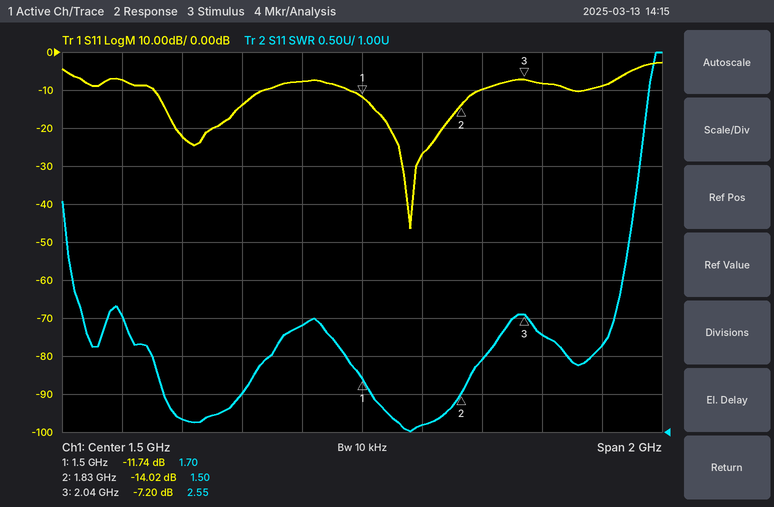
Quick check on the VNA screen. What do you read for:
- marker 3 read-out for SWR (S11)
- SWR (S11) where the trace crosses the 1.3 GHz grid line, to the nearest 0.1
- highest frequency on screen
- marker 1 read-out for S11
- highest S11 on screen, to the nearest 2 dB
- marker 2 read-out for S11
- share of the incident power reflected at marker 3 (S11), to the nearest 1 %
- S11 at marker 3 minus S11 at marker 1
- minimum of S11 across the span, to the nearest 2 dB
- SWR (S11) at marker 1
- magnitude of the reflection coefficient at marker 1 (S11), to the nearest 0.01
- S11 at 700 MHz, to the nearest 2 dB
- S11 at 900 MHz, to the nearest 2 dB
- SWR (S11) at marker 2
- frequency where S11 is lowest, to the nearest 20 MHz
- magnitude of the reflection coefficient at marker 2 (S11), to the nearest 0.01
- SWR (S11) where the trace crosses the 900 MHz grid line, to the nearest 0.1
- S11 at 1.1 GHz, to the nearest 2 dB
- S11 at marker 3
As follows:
2.55
2.4
2.5 GHz
-11.74 dB
-2 dB
-14.02 dB
19 %
4.54 dB
-46 dB
1.70
0.26
-8 dB
-22 dB
1.50
1.66 GHz
0.20
1.2
-14 dB
-7.20 dB
